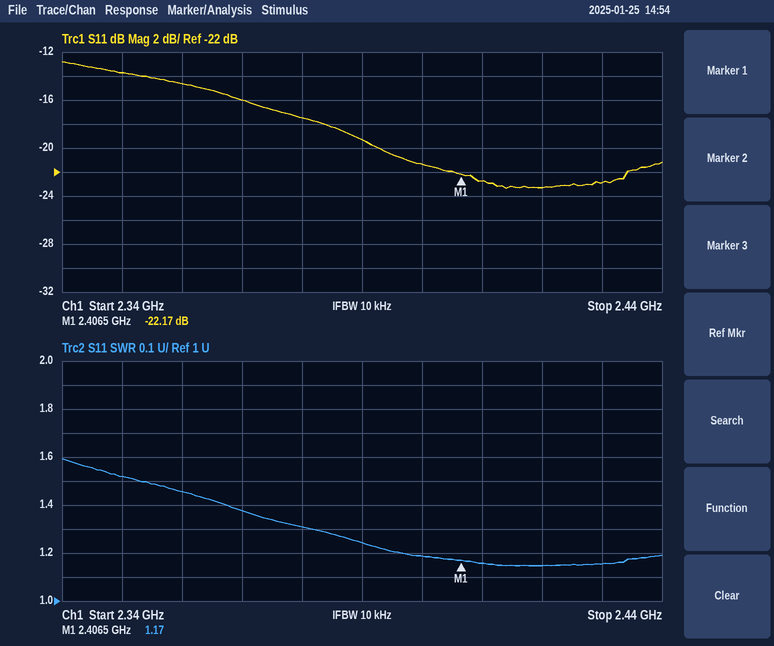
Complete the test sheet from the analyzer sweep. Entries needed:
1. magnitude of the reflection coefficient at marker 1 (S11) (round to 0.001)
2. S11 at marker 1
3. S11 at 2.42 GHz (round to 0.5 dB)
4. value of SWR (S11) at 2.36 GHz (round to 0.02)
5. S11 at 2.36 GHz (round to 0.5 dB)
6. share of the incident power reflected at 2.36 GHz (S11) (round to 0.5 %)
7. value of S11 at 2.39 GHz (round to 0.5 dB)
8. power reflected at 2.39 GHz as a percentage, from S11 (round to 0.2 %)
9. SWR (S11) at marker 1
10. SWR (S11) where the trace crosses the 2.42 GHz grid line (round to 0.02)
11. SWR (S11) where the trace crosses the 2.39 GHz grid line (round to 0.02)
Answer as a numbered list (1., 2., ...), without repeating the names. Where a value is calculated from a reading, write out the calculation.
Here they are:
1. 10^(-22.17/20) ≈ 0.078
2. -22.17 dB
3. -23.5 dB
4. 1.46
5. -14.5 dB
6. 10^(-14.5/10) ≈ 3.5 %
7. -19.5 dB
8. 10^(-19.5/10) ≈ 1.12 %, so 1.2 % to the nearest 0.2 %
9. 1.17
10. 1.14
11. 1.24
